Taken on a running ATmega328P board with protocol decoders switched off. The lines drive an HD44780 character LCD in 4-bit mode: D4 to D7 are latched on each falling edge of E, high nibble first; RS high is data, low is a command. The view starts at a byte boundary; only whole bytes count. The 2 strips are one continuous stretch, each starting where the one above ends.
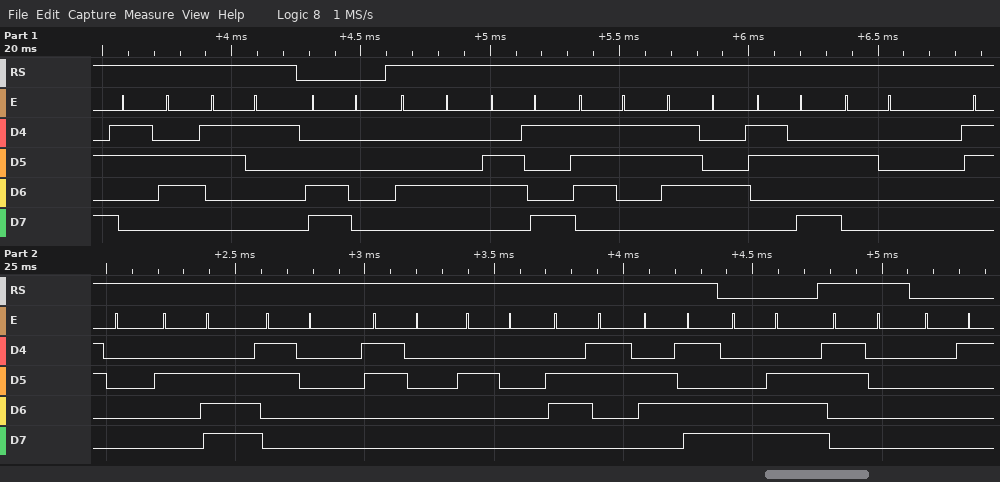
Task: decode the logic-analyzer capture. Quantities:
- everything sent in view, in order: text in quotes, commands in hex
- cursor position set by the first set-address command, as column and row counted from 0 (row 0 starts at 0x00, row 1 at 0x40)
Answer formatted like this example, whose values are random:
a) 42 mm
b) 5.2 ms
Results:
a) "61" 0xC0 "Dist: 0.00 cm" 0xCE "0" 0x01
b) column 0, row 1
